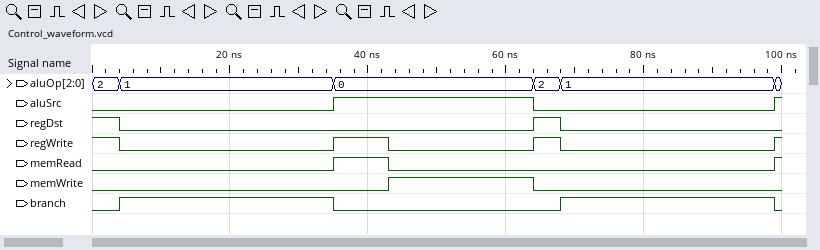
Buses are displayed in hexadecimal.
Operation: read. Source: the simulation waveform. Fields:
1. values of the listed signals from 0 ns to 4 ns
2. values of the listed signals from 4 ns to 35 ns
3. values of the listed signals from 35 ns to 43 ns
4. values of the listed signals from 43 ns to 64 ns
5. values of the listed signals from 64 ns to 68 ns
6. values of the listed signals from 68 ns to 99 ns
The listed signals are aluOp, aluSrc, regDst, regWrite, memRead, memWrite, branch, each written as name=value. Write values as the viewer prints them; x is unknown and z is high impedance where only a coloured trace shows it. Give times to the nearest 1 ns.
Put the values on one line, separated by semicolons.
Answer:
aluOp=2, aluSrc=0, regDst=1, regWrite=1, memRead=0, memWrite=0, branch=0; aluOp=1, aluSrc=0, regDst=0, regWrite=0, memRead=0, memWrite=0, branch=1; aluOp=0, aluSrc=1, regDst=0, regWrite=1, memRead=1, memWrite=0, branch=0; aluOp=0, aluSrc=1, regDst=0, regWrite=0, memRead=0, memWrite=1, branch=0; aluOp=2, aluSrc=0, regDst=1, regWrite=1, memRead=0, memWrite=0, branch=0; aluOp=1, aluSrc=0, regDst=0, regWrite=0, memRead=0, memWrite=0, branch=1
